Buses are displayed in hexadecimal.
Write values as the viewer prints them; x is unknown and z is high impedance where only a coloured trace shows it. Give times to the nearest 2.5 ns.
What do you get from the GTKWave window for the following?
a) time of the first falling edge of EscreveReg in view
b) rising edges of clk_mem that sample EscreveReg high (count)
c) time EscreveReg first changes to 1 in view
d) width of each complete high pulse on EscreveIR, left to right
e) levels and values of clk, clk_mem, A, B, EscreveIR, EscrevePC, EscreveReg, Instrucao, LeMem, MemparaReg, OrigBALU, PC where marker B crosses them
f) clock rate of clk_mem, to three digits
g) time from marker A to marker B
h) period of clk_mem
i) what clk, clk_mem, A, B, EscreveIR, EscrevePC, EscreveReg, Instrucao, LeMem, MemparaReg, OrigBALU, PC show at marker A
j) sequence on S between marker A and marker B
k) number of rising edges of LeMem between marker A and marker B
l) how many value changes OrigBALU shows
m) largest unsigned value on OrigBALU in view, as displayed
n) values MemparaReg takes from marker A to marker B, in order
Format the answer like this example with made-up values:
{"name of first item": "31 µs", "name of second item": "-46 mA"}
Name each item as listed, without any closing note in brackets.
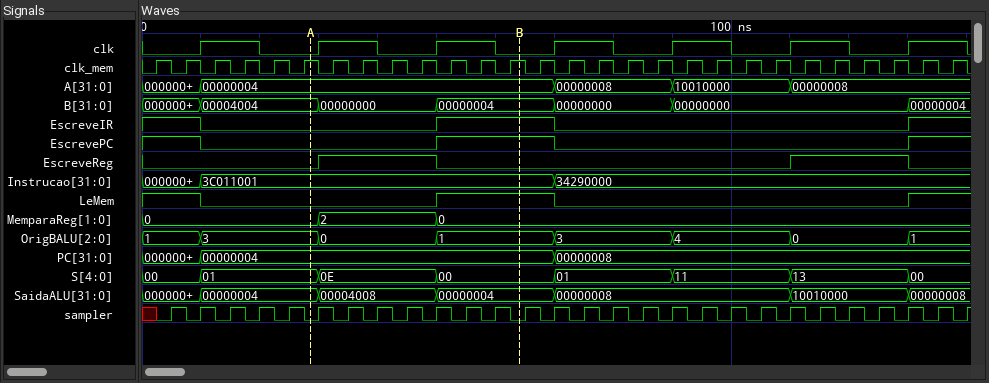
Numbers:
{"time of the first falling edge of EscreveReg in view": "50 ns", "rising edges of clk_mem that sample EscreveReg high": "8", "time EscreveReg first changes to 1 in view": "30 ns", "width of each complete high pulse on EscreveIR, left to right": "20 ns", "levels and values of clk, clk_mem, A, B, EscreveIR, EscrevePC, EscreveReg, Instrucao, LeMem, MemparaReg, OrigBALU, PC where marker B crosses them": "clk=0, clk_mem=1, A=00000004, B=00000004, EscreveIR=1, EscrevePC=1, EscreveReg=0, Instrucao=3C011001, LeMem=1, MemparaReg=0, OrigBALU=1, PC=00000004", "clock rate of clk_mem, to three digits": "200 MHz", "time from marker A to marker B": "35 ns", "period of clk_mem": "5 ns", "what clk, clk_mem, A, B, EscreveIR, EscrevePC, EscreveReg, Instrucao, LeMem, MemparaReg, OrigBALU, PC show at marker A": "clk=0, clk_mem=1, A=00000004, B=00004004, EscreveIR=0, EscrevePC=0, EscreveReg=0, Instrucao=3C011001, LeMem=0, MemparaReg=0, OrigBALU=3, PC=00000004", "sequence on S between marker A and marker B": "01, 0E, 00", "number of rising edges of LeMem between marker A and marker B": "1", "how many value changes OrigBALU shows": "7", "largest unsigned value on OrigBALU in view, as displayed": "4", "values MemparaReg takes from marker A to marker B, in order": "0, 2, 0"}
